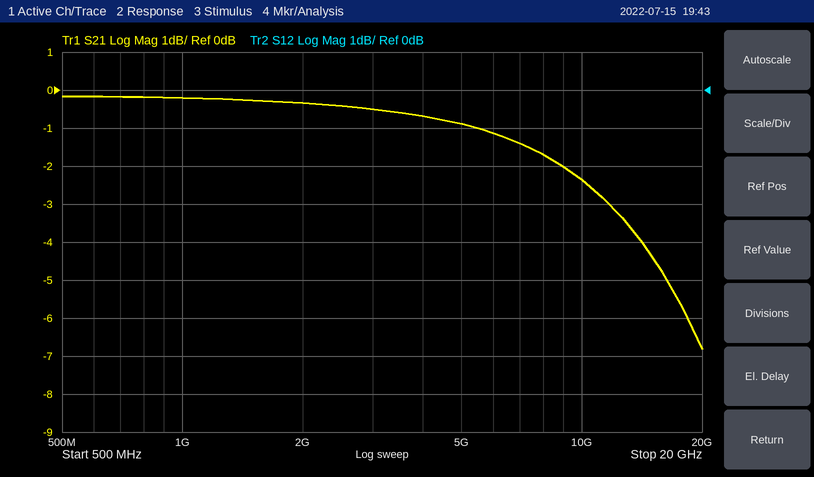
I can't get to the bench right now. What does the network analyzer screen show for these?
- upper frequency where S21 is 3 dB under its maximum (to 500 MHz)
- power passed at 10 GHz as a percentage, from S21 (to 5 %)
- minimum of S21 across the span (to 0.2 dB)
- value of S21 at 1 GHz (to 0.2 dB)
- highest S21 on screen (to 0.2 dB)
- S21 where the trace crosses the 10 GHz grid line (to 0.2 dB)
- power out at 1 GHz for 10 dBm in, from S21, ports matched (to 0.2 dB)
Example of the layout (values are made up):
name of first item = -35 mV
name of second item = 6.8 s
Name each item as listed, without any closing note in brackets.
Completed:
upper frequency where S21 is 3 dB under its maximum = 12.0 GHz
power passed at 10 GHz as a percentage, from S21 = 60 %
minimum of S21 across the span = -6.8 dB
value of S21 at 1 GHz = -0.2 dB
highest S21 on screen = -0.2 dB
S21 where the trace crosses the 10 GHz grid line = -2.4 dB
power out at 1 GHz for 10 dBm in, from S21, ports matched = 9.8 dBm
